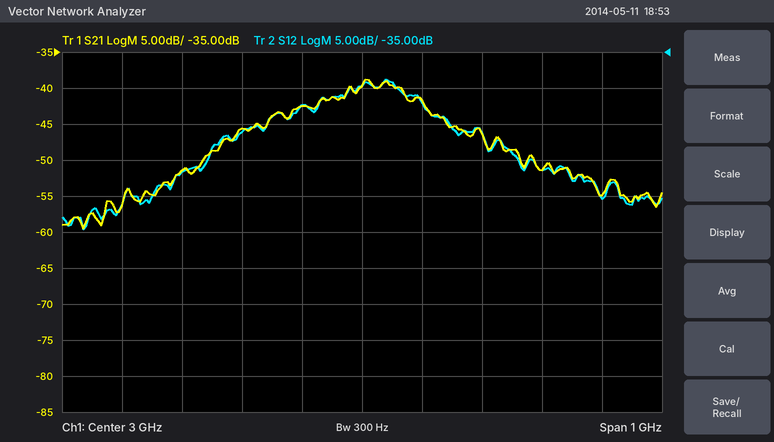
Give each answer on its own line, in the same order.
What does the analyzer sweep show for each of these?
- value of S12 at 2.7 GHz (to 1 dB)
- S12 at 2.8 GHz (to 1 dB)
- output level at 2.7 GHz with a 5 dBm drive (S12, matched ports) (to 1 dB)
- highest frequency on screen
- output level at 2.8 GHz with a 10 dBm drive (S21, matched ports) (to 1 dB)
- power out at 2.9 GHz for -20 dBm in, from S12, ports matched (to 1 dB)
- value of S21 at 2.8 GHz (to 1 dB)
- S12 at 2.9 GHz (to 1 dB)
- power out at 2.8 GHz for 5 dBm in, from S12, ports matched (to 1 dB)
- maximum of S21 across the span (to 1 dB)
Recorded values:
-52 dB
-46 dB
-47 dBm
3.5 GHz
-36 dBm
-62 dBm
-46 dB
-42 dB
-41 dBm
-39 dB
